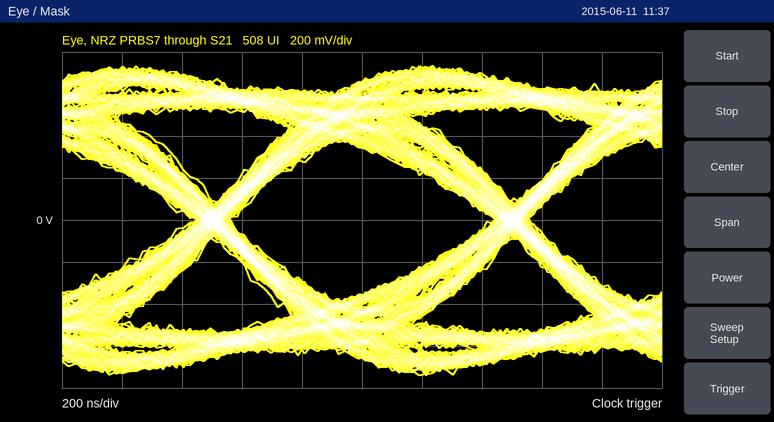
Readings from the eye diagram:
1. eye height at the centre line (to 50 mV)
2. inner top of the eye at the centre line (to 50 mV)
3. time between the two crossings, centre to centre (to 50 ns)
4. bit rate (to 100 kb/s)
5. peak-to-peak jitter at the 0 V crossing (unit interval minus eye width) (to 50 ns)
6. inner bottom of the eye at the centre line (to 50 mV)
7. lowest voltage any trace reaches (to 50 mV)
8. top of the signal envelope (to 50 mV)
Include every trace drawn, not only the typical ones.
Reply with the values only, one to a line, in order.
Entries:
700 mV
350 mV
1.00 µs
1.0 Mb/s
100 ns
-350 mV
-750 mV
750 mV
